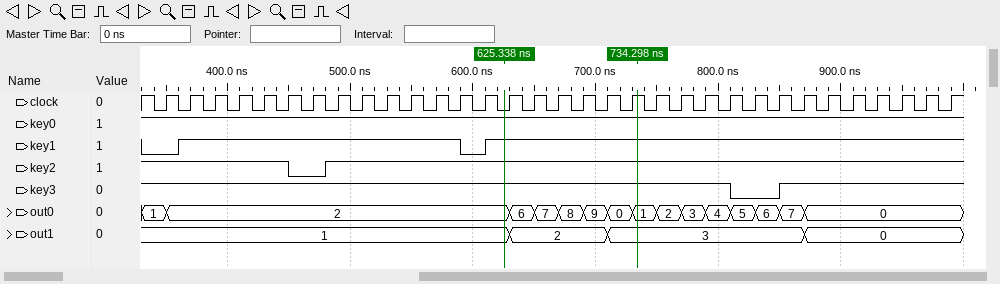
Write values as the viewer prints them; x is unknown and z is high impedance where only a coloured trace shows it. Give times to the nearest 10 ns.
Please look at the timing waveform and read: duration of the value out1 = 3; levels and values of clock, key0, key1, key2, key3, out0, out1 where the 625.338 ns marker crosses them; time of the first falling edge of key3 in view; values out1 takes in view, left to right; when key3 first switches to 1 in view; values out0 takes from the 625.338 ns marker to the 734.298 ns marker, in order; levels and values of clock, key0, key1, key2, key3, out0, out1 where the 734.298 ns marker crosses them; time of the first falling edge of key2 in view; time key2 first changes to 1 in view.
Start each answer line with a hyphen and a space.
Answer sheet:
- 160 ns
- clock=0, key0=1, key1=1, key2=1, key3=1, out0=2, out1=1
- 810 ns
- 1, 2, 3, 0
- 850 ns
- 2, 6, 7, 8, 9, 0, 1
- clock=1, key0=1, key1=1, key2=1, key3=1, out0=1, out1=3
- 450 ns
- 480 ns
